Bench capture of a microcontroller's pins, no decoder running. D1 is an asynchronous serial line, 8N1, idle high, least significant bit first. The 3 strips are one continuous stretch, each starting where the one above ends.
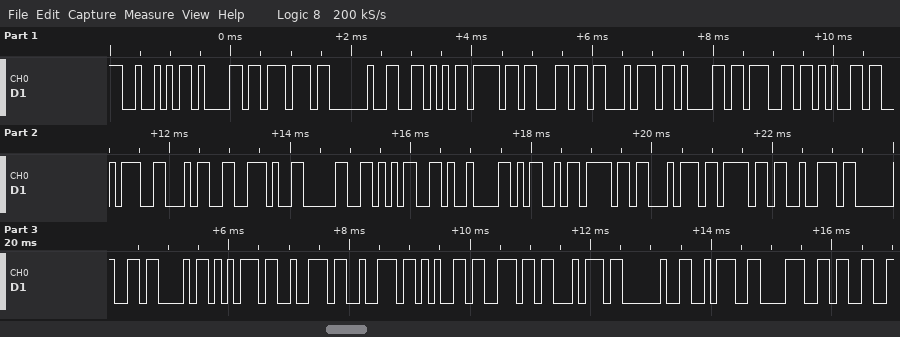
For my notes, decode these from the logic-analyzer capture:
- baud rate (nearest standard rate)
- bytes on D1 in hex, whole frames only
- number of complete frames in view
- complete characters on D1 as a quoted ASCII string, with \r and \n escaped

9600 baud
52 61 77 20 56 6F 6C 74 61 67 65 3A 34 2E 30 35 09 4D 6F 74 6F 72 20 43 75 72 72 65 6E 74 20 3A 38 33
34
"Raw Voltage:4.05\tMotor Current :83"
